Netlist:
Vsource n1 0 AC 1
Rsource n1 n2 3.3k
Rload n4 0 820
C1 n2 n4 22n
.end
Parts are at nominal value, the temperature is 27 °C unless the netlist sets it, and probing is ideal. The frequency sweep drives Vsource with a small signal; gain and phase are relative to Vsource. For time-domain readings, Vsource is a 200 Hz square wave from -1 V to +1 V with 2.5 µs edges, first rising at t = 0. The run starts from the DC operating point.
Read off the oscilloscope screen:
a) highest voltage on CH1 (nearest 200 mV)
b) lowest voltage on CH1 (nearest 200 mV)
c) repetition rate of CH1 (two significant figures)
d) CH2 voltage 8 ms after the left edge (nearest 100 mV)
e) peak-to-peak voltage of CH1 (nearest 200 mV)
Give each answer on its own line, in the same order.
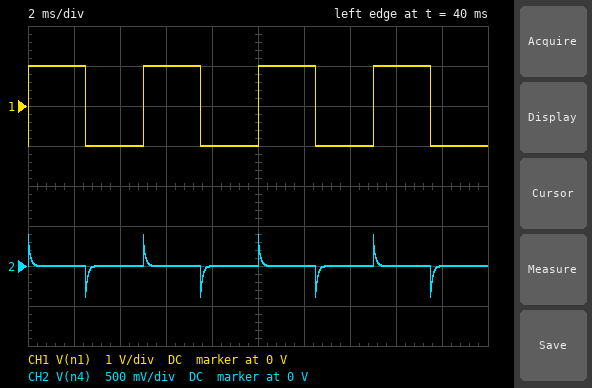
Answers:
1.0 V
-1.0 V
200 Hz
0 V
2.0 V
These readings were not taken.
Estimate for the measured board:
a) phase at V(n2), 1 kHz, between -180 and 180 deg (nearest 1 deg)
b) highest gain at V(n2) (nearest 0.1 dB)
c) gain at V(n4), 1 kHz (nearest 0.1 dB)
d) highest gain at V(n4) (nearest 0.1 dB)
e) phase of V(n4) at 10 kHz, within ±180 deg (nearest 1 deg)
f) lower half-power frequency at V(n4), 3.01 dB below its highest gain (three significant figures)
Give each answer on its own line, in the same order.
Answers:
-23 deg
0 dB
-20.1 dB
-14.0 dB
10 deg
1.76 kHz
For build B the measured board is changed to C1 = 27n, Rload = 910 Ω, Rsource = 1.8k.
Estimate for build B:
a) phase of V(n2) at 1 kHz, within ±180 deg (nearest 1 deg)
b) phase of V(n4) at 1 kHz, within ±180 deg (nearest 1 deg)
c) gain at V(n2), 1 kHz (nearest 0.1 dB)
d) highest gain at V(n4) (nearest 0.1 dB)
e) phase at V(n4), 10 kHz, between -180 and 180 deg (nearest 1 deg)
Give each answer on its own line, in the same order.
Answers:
-16 deg
65 deg
-0.7 dB
-9.5 dB
12 deg
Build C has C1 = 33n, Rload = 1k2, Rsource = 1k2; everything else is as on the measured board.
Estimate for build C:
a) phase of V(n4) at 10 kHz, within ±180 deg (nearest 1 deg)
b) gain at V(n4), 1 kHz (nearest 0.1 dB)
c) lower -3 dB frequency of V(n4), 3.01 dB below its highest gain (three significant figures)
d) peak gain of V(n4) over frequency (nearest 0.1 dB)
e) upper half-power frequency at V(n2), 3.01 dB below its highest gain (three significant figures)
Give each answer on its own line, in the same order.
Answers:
11 deg
-13.0 dB
2.01 kHz
-6.0 dB
2.84 kHz
